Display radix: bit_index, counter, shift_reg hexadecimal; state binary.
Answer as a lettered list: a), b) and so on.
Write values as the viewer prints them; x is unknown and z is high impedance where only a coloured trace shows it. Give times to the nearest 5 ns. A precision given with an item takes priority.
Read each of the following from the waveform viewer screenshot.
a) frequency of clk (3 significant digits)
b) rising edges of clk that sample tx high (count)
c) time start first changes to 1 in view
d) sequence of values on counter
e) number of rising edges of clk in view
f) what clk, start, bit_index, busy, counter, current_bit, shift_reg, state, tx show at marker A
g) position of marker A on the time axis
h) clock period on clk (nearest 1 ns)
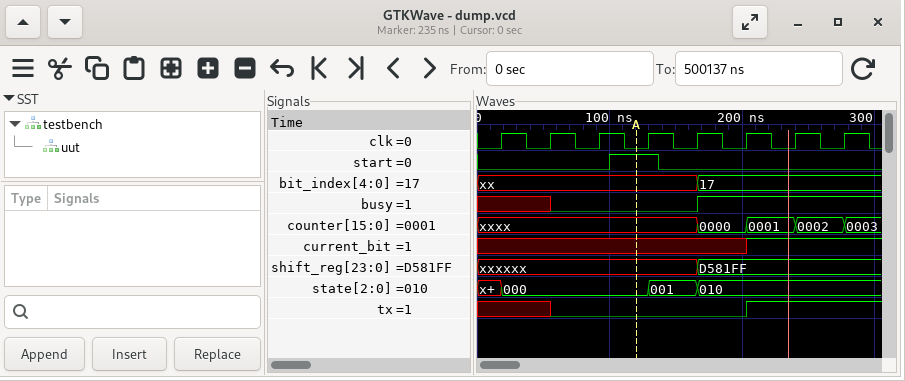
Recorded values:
a) 27.0 MHz
b) 2
c) 100 ns
d) xxxx, 0000, 0001, 0002, 0003
e) 8
f) clk=0, start=1, bit_index=xx, busy=0, counter=xxxx, current_bit=x, shift_reg=xxxxxx, state=000, tx=0
g) 120 ns
h) 37 ns
